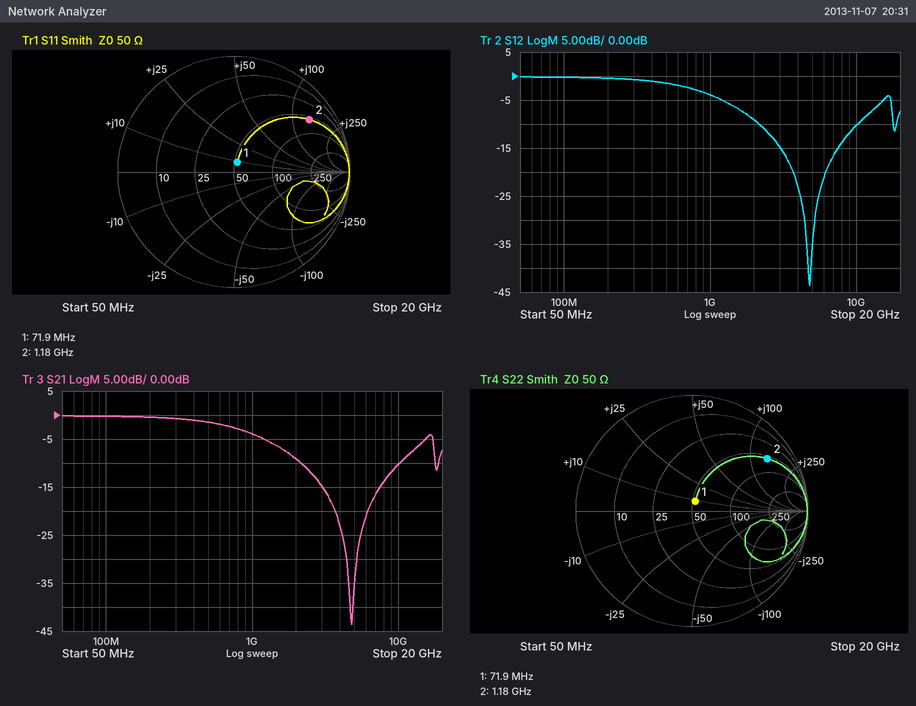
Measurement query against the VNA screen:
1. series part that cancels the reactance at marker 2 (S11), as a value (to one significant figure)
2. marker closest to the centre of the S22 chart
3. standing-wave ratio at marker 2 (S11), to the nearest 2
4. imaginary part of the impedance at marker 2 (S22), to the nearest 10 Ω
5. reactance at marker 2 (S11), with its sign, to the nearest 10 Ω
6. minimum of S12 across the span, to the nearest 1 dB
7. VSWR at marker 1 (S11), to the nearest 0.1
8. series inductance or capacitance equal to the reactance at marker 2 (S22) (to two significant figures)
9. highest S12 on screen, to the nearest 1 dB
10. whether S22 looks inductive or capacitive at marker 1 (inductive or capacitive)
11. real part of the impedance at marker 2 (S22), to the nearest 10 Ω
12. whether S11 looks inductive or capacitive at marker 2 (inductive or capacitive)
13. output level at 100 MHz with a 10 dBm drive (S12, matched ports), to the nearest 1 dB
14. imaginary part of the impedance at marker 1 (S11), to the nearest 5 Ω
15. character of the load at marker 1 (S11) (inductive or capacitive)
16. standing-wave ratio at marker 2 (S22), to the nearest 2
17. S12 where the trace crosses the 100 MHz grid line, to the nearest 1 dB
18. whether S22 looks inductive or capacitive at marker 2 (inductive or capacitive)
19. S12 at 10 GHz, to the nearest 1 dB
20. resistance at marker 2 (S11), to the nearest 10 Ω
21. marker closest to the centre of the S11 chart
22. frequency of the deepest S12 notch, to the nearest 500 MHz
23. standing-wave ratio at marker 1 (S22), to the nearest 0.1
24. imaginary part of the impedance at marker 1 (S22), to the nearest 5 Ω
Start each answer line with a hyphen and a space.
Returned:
- 1.0 pF
- marker 1
- 8
- +140 Ω
- +140 Ω
- -44 dB
- 1.2
- 19 nH
- 0 dB
- inductive
- 60 Ω
- inductive
- 10 dBm
- +10 Ω
- inductive
- 8
- 0 dB
- inductive
- -10 dB
- 60 Ω
- marker 1
- 5.0 GHz
- 1.2
- +10 Ω
